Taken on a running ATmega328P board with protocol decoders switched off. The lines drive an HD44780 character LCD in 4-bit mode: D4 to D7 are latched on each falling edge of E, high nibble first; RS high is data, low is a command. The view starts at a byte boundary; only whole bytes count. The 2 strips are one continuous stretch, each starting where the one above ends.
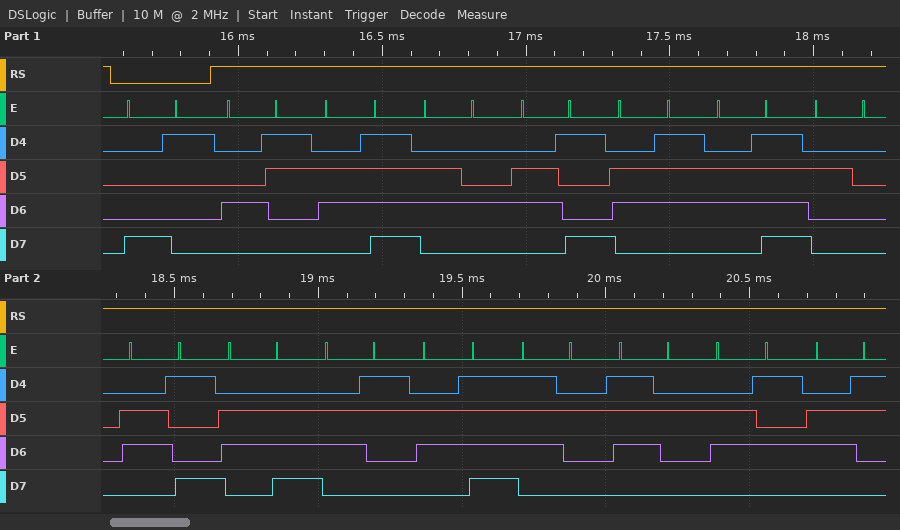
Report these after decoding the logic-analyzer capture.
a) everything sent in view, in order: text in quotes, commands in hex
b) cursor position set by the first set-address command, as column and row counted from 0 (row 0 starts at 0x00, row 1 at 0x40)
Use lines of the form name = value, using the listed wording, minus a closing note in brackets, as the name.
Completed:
everything sent in view, in order: text in quotes, commands in hex = 0x81 "Codigo incorrec"
cursor position set by the first set-address command, as column and row counted from 0 = column 1, row 0
